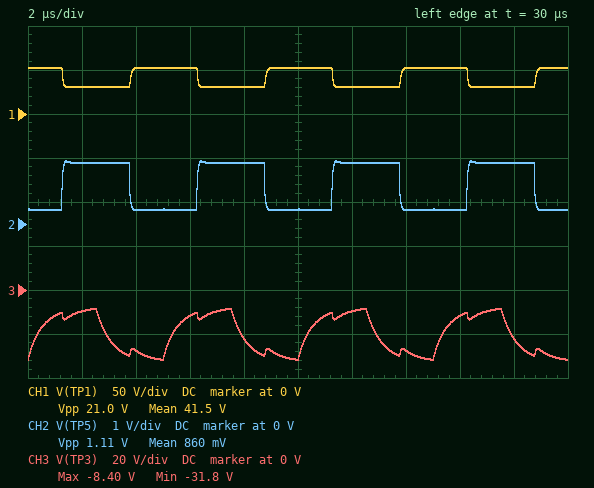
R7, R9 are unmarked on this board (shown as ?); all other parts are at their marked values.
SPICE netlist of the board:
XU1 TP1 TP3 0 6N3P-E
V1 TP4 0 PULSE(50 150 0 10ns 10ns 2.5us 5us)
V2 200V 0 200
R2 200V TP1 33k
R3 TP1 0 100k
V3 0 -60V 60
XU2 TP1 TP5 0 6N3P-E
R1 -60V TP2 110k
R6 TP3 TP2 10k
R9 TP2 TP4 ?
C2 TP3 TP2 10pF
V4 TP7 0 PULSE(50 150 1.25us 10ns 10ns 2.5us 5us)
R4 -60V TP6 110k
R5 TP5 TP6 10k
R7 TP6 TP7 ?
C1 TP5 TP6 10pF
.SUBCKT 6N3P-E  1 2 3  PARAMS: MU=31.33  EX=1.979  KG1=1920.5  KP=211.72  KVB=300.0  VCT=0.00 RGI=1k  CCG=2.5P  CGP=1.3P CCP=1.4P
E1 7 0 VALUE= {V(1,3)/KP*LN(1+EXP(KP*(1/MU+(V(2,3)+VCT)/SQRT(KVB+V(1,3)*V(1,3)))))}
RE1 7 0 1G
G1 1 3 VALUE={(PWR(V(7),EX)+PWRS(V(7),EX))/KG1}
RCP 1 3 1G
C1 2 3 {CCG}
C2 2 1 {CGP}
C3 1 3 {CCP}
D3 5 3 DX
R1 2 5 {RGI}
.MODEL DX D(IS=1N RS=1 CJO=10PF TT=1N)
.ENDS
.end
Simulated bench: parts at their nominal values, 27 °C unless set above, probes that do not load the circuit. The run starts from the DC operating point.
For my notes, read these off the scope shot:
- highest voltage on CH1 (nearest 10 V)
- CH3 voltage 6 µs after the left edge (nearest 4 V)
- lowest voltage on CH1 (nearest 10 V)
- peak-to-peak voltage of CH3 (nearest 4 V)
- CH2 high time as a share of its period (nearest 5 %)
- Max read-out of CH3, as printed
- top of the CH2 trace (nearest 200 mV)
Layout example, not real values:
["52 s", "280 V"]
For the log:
["50 V", "-12 V", "30 V", "24 V", "50 %", "-8.40 V", "1.4 V"]
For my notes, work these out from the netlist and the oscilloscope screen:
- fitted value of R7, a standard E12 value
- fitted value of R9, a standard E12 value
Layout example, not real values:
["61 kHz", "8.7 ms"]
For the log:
["82 kΩ", "330 kΩ"]
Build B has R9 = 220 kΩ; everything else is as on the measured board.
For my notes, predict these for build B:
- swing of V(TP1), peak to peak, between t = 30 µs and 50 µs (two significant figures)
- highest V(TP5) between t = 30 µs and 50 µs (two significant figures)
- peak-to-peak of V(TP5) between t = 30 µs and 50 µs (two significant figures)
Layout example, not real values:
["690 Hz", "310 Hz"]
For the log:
["26 V", "1.5 V", "1.4 V"]
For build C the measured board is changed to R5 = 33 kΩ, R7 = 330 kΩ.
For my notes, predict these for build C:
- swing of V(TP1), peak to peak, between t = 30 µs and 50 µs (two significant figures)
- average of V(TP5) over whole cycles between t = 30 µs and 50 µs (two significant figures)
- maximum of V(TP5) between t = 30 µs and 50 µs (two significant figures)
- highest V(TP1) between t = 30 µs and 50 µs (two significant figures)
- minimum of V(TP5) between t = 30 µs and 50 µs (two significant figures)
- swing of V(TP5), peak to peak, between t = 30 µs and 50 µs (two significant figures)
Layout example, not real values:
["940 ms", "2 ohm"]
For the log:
["2.0 V", "-20 V", "-8.6 V", "150 V", "-32 V", "23 V"]
